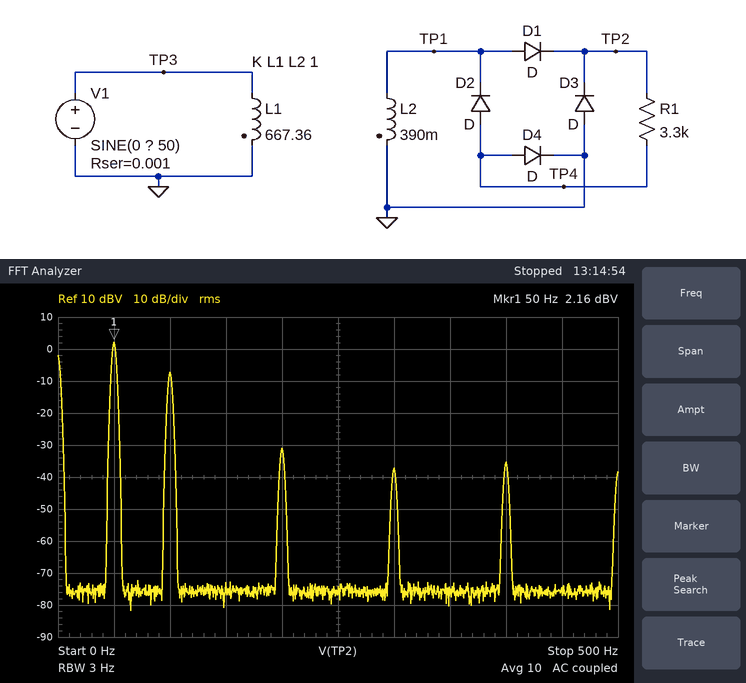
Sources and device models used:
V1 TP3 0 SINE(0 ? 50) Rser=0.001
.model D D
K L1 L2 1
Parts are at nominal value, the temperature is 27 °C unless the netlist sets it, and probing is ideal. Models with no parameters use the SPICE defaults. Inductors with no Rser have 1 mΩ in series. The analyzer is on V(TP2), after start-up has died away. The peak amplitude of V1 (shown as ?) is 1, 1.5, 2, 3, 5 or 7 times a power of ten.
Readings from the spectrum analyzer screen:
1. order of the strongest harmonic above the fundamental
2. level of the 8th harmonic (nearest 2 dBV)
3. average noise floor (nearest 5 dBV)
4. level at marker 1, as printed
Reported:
2
-36 dBV
-75 dBV
2.16 dBV
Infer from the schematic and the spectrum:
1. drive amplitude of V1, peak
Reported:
150 V
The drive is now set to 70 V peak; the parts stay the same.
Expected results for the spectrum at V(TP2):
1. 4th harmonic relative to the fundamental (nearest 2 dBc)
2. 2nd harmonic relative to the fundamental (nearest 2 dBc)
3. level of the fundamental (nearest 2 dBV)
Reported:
-26 dBc
-16 dBc
-4 dBV
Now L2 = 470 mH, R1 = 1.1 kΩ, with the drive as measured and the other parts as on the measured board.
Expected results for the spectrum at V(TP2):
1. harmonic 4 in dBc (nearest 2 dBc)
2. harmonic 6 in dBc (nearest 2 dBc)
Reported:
-32 dBc
-42 dBc
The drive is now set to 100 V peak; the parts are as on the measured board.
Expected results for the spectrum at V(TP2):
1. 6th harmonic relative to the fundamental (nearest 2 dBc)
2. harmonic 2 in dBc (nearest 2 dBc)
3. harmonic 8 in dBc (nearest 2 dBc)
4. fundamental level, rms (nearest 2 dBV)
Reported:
-32 dBc
-12 dBc
-40 dBc
-2 dBV
